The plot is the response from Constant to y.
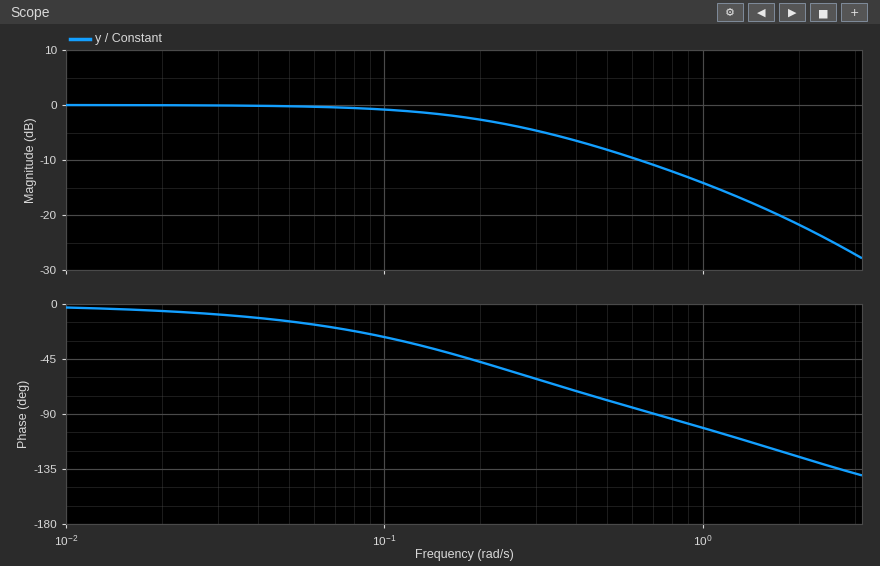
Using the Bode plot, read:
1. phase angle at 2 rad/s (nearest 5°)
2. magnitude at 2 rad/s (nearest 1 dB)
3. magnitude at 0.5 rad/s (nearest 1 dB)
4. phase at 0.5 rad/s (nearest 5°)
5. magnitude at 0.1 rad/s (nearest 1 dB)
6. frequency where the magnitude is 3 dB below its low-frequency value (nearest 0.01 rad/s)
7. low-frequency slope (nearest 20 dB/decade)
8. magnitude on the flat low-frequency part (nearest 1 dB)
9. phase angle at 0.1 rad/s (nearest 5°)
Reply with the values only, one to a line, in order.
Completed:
-125°
-22 dB
-8 dB
-80°
-1 dB
0.22 rad/s
0 dB/decade
0 dB
-25°
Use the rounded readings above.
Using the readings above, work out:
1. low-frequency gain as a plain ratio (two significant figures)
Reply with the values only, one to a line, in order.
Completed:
1.0
